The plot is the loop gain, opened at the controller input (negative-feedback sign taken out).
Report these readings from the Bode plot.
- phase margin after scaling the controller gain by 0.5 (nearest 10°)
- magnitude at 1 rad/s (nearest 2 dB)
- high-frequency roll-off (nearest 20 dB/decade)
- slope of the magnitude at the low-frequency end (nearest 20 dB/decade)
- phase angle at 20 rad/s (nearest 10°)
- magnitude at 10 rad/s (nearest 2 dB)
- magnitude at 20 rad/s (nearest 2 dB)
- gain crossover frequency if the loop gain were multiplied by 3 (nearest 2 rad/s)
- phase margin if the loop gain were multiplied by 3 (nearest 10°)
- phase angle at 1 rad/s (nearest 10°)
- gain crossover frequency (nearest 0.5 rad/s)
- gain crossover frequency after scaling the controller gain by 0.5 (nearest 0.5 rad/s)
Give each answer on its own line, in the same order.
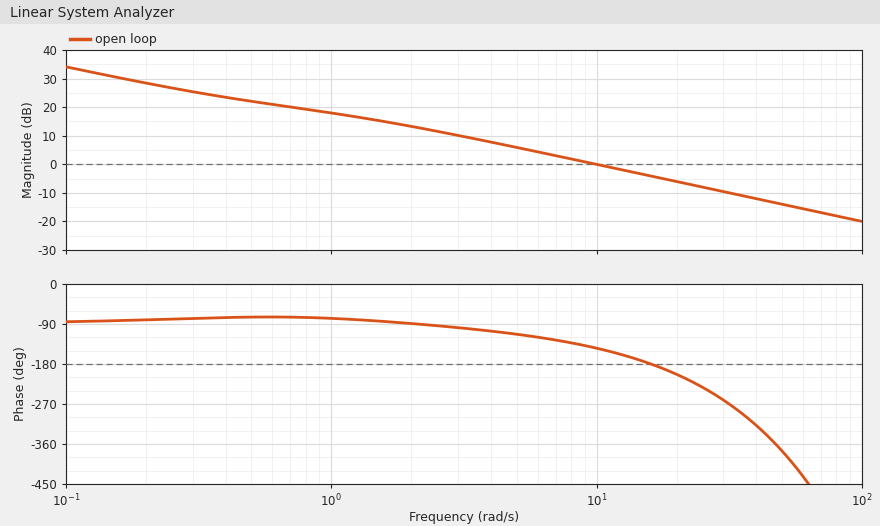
70°
18 dB
-20 dB/decade
-20 dB/decade
-200°
0 dB
-6 dB
30 rad/s
-80°
-80°
10.0 rad/s
5.0 rad/s
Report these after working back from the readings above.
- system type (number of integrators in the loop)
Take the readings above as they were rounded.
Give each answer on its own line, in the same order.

1
